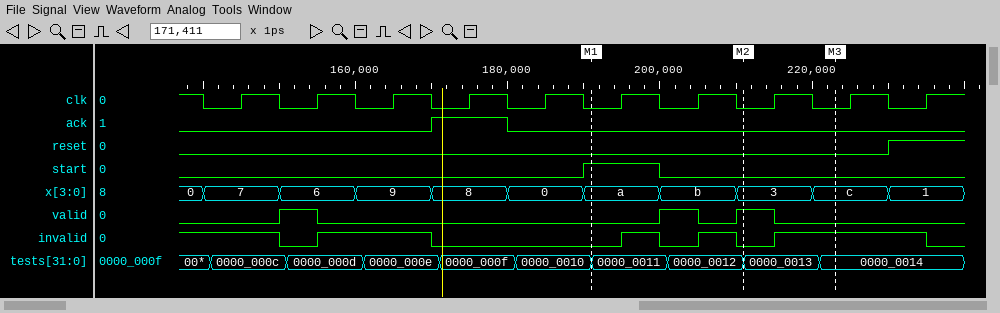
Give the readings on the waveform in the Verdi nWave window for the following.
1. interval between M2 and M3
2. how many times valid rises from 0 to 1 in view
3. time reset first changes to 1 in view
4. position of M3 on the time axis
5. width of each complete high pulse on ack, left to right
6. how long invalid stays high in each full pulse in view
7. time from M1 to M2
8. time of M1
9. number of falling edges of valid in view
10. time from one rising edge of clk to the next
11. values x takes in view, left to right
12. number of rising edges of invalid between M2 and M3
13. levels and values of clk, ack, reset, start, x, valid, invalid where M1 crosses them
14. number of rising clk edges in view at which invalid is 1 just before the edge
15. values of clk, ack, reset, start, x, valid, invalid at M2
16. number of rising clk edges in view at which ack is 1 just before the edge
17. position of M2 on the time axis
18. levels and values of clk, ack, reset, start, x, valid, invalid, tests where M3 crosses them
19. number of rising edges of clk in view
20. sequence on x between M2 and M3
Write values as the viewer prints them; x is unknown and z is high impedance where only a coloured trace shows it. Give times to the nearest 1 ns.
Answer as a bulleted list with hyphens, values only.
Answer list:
- 12 ns
- 3
- 230 ns
- 223 ns
- 10 ns
- 15 ns, 5 ns, 5 ns, 20 ns
- 20 ns
- 191 ns
- 3
- 10 ns
- 0, 7, 6, 9, 8, 0, a, b, 3, c, 1
- 1
- clk=0, ack=0, reset=0, start=1, x=a, valid=0, invalid=0
- 4
- clk=0, ack=0, reset=0, start=0, x=3, valid=1, invalid=0
- 1
- 211 ns
- clk=0, ack=0, reset=0, start=0, x=c, valid=0, invalid=1, tests=0000_0014
- 10
- 3, c
